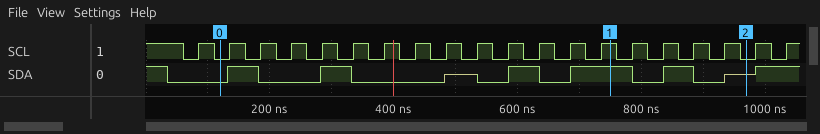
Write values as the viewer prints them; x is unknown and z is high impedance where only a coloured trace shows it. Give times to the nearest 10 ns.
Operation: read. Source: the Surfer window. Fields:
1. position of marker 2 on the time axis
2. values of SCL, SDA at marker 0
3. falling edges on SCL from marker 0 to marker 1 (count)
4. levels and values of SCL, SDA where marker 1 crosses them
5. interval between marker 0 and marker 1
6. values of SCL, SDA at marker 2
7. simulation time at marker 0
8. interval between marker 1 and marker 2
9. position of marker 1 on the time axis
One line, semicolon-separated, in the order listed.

970 ns; SCL=0, SDA=0; 12; SCL=1, SDA=1; 630 ns; SCL=0, SDA=z; 120 ns; 220 ns; 750 ns
